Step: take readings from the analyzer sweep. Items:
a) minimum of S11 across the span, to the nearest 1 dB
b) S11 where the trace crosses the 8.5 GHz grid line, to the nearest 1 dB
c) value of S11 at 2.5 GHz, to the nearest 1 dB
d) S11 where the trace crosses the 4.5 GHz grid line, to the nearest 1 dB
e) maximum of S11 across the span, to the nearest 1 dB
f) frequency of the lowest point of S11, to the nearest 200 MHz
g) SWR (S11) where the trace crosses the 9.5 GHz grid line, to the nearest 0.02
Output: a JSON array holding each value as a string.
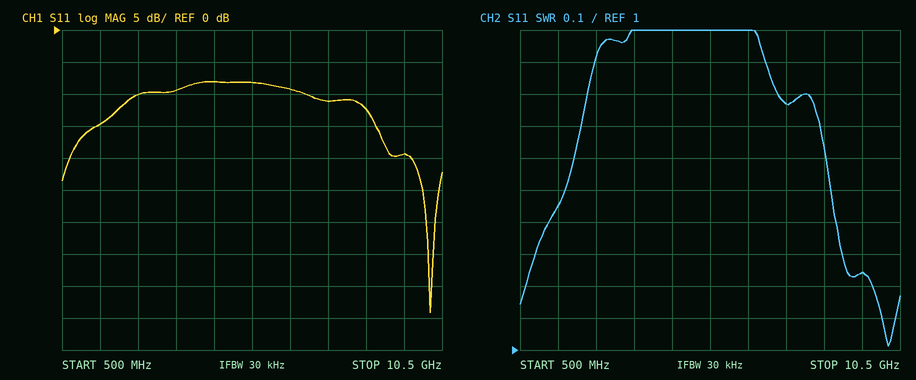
["-44 dB", "-12 dB", "-10 dB", "-8 dB", "-8 dB", "10.2 GHz", "1.24"]
